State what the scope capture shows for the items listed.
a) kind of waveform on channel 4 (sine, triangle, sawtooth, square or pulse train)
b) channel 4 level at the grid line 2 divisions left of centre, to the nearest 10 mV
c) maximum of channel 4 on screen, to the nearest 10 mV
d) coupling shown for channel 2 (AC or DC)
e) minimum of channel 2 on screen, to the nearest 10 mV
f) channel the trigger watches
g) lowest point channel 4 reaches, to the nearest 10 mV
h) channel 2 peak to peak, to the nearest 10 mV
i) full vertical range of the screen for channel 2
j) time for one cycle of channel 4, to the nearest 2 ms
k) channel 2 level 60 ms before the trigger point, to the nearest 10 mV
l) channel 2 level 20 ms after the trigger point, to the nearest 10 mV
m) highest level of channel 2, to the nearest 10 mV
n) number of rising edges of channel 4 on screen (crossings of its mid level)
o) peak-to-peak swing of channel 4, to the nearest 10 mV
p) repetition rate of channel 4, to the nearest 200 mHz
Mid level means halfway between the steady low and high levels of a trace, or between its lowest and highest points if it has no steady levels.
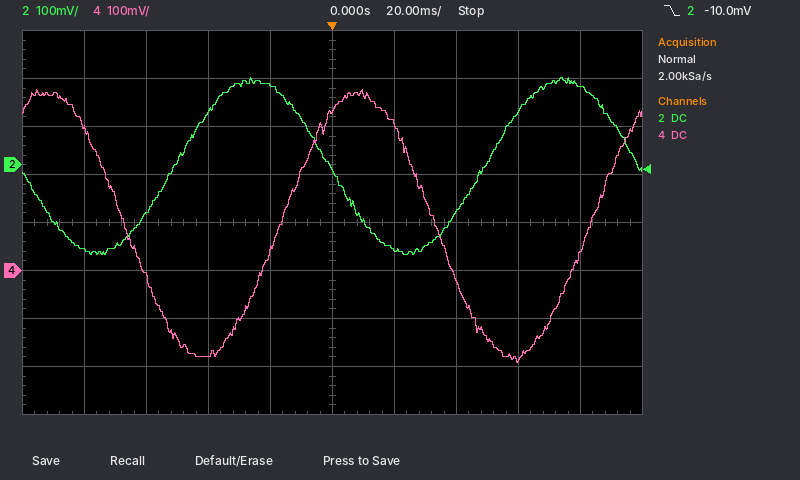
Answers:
sine
-180 mV
380 mV
DC
-190 mV
channel 2
-190 mV
370 mV
800 mV
100 ms
-100 mV
-180 mV
180 mV
2
570 mV
10.0 Hz
